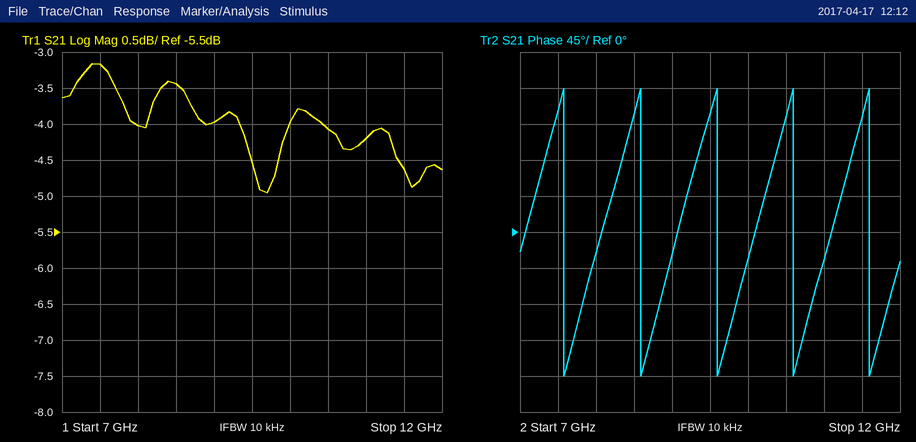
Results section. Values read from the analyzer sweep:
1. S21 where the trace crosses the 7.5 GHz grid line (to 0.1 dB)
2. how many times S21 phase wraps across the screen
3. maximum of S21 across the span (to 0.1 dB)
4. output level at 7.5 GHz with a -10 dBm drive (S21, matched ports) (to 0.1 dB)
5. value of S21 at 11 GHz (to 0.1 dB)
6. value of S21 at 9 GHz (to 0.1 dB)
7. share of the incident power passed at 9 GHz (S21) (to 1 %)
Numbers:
-3.2 dB
5
-3.2 dB
-13.2 dBm
-4.2 dB
-4.0 dB
40 %
